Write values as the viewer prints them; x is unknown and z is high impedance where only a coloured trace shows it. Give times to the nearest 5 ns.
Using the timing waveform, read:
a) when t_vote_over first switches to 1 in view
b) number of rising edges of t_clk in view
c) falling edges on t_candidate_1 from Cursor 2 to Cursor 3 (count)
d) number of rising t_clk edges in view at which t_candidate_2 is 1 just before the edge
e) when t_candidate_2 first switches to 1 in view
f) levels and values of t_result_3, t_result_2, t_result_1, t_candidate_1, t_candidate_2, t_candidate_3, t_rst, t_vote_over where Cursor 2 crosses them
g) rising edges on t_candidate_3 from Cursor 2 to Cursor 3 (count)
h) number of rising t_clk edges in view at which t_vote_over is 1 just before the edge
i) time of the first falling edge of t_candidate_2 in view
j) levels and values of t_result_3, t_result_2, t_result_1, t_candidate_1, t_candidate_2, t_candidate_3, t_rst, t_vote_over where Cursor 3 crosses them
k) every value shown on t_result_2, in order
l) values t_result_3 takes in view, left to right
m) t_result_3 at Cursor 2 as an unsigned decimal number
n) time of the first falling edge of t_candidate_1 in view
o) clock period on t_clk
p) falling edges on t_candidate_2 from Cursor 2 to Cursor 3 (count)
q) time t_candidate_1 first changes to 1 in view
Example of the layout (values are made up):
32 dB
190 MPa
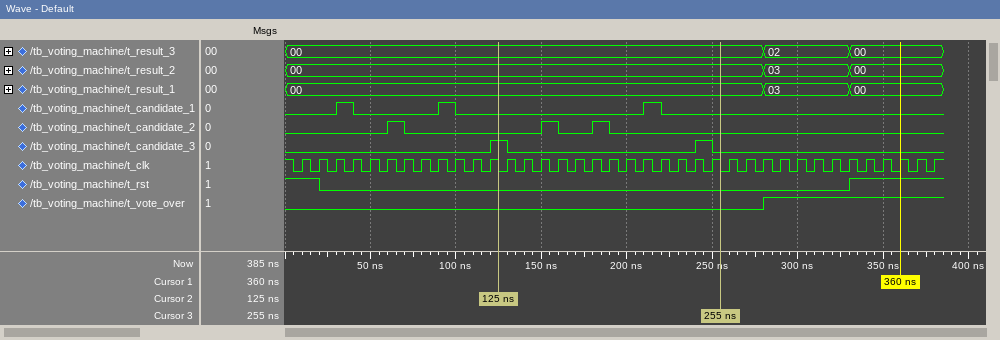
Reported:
280 ns
38
1
3
60 ns
t_result_3=00, t_result_2=00, t_result_1=00, t_candidate_1=0, t_candidate_2=0, t_candidate_3=1, t_rst=0, t_vote_over=0
1
10
70 ns
t_result_3=00, t_result_2=00, t_result_1=00, t_candidate_1=0, t_candidate_2=0, t_candidate_3=0, t_rst=0, t_vote_over=0
00, 03, 00
00, 02, 00
0
40 ns
10 ns
2
30 ns
